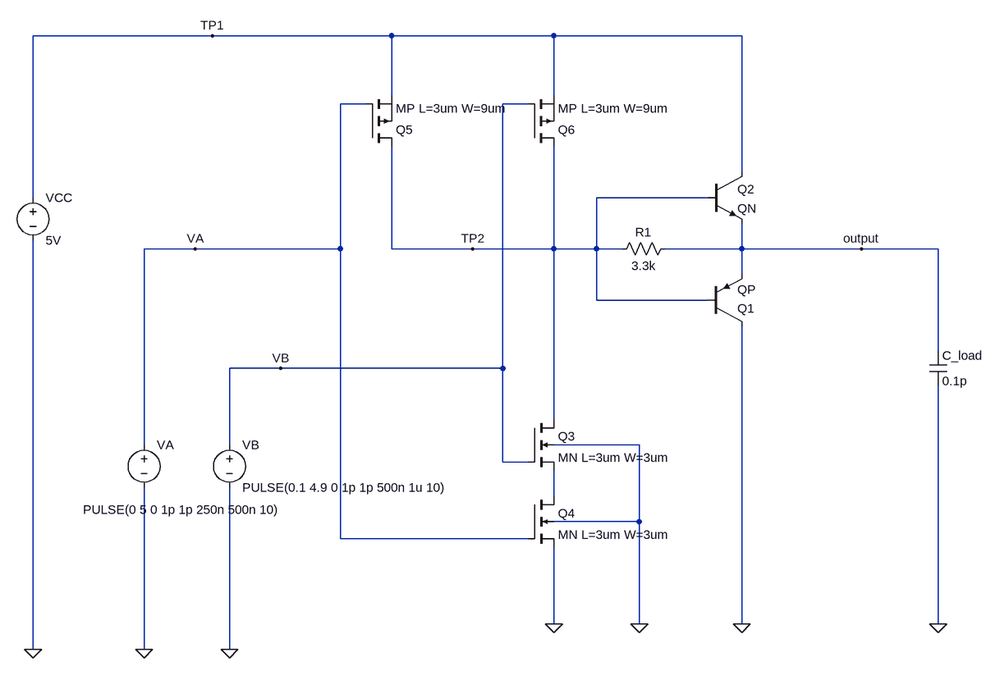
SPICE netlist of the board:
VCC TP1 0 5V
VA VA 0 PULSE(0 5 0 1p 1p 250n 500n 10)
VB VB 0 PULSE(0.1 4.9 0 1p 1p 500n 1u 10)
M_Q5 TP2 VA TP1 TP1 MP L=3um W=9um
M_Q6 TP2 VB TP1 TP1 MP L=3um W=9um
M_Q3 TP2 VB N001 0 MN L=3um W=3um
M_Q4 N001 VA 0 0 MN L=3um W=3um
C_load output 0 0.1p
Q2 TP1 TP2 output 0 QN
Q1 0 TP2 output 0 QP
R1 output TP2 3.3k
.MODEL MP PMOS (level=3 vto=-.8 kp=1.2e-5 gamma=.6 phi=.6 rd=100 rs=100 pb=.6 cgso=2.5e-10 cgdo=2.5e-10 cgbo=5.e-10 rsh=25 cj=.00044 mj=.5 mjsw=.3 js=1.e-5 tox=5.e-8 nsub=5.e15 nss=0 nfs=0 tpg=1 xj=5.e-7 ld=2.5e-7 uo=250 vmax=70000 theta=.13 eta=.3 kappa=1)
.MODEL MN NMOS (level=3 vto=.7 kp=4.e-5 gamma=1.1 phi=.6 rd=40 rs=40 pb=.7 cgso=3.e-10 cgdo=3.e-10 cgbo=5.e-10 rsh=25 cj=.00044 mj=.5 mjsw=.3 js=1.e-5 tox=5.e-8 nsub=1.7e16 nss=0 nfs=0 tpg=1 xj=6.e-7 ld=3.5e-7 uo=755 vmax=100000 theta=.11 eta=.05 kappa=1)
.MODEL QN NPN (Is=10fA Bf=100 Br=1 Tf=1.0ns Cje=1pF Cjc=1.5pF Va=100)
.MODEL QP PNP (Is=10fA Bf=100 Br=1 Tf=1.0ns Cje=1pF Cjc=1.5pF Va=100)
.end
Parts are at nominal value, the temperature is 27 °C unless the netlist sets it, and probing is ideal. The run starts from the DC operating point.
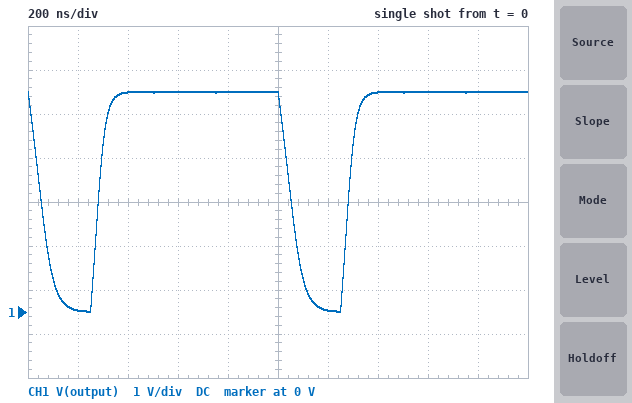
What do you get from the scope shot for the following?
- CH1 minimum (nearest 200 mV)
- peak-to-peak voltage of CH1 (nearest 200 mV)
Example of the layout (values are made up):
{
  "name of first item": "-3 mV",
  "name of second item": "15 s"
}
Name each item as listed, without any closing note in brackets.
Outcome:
{
  "CH1 minimum": "0 V",
  "peak-to-peak voltage of CH1": "5.0 V"
}
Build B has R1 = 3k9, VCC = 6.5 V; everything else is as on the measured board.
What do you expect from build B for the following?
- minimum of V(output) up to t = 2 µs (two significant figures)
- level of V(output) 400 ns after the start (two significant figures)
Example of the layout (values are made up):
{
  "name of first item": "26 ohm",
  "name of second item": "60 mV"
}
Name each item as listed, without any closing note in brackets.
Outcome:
{
  "minimum of V(output) up to t = 2 µs": "440 mV",
  "level of V(output) 400 ns after the start": "6.5 V"
}
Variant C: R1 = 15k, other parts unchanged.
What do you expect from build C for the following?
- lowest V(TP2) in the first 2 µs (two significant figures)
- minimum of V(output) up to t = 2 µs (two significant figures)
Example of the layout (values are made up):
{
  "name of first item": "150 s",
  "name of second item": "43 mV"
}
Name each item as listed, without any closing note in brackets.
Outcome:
{
  "lowest V(TP2) in the first 2 µs": "2.0 mV",
  "minimum of V(output) up to t = 2 µs": "4.2 mV"
}
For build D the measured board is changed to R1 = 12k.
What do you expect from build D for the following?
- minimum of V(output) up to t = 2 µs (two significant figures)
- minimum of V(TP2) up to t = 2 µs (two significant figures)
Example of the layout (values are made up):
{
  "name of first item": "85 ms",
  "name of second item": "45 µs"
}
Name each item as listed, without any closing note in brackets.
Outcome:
{
  "minimum of V(output) up to t = 2 µs": "3.2 mV",
  "minimum of V(TP2) up to t = 2 µs": "2.0 mV"
}
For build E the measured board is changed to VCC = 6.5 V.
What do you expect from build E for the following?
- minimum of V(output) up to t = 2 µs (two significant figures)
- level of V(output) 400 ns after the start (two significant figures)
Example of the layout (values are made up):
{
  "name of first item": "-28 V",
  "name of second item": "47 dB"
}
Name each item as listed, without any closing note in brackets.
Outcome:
{
  "minimum of V(output) up to t = 2 µs": "440 mV",
  "level of V(output) 400 ns after the start": "6.5 V"
}
